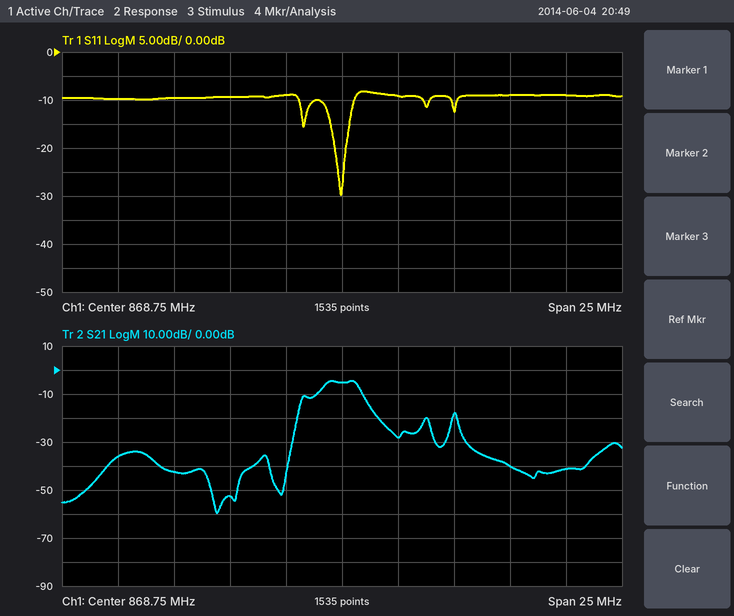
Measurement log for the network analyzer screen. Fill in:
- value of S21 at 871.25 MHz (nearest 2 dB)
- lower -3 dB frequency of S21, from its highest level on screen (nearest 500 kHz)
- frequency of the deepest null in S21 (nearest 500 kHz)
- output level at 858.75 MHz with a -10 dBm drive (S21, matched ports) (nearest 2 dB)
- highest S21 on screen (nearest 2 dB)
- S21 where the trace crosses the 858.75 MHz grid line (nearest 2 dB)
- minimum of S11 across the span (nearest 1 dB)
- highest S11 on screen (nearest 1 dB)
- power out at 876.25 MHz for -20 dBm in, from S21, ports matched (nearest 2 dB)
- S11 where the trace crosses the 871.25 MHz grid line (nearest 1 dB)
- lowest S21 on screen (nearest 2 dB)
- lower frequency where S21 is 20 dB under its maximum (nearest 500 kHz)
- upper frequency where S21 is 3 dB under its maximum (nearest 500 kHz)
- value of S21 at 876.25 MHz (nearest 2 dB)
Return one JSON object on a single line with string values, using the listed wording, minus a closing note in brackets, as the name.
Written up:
{"value of S21 at 871.25 MHz": "-28 dB", "lower -3 dB frequency of S21, from its highest level on screen": "868.0 MHz", "frequency of the deepest null in S21": "863.0 MHz", "output level at 858.75 MHz with a -10 dBm drive (S21, matched ports)": "-46 dBm", "highest S21 on screen": "-4 dB", "S21 where the trace crosses the 858.75 MHz grid line": "-36 dB", "minimum of S11 across the span": "-30 dB", "highest S11 on screen": "-8 dB", "power out at 876.25 MHz for -20 dBm in, from S21, ports matched": "-60 dBm", "S11 where the trace crosses the 871.25 MHz grid line": "-9 dB", "lowest S21 on screen": "-60 dB", "lower frequency where S21 is 20 dB under its maximum": "866.5 MHz", "upper frequency where S21 is 3 dB under its maximum": "869.5 MHz", "value of S21 at 876.25 MHz": "-40 dB"}
